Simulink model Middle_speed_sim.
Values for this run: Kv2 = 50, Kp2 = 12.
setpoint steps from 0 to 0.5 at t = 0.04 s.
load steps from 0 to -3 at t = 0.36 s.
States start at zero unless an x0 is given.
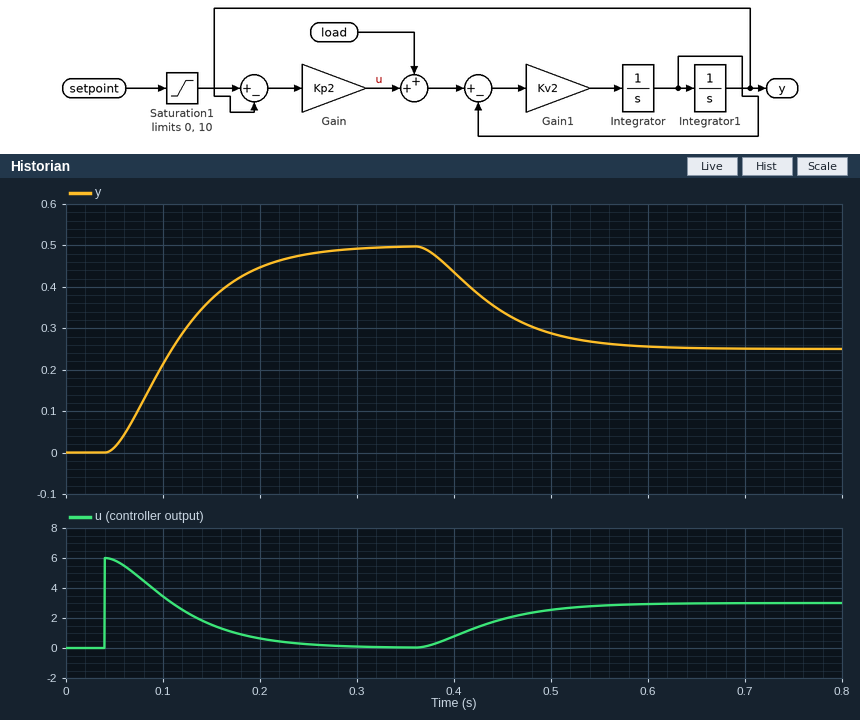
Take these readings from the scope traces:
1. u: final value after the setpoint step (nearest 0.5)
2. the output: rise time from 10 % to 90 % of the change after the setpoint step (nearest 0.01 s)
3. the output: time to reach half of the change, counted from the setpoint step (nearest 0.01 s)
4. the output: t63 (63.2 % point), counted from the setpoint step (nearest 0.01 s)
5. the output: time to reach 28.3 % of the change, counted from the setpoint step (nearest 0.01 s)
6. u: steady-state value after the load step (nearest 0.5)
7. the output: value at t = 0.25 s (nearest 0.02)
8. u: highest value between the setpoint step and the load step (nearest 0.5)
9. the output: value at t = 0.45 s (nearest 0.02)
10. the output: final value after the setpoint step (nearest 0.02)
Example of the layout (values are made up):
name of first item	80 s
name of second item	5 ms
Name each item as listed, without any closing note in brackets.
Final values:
u: final value after the setpoint step	0.0
the output: rise time from 10 % to 90 % of the change after the setpoint step	0.14 s
the output: time to reach half of the change, counted from the setpoint step	0.07 s
the output: t63 (63.2 % point), counted from the setpoint step	0.09 s
the output: time to reach 28.3 % of the change, counted from the setpoint step	0.04 s
u: steady-state value after the load step	3.0
the output: value at t = 0.25 s	0.48
u: highest value between the setpoint step and the load step	6.0
the output: value at t = 0.45 s	0.34
the output: final value after the setpoint step	0.50
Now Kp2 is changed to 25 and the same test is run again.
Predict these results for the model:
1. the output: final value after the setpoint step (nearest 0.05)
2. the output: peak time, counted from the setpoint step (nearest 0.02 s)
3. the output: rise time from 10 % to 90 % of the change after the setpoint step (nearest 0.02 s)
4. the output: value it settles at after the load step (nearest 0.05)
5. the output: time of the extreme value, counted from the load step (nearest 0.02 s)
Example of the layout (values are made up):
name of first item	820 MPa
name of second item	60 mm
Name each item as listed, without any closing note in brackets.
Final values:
the output: final value after the setpoint step	0.50
the output: peak time, counted from the setpoint step	0.12 s
the output: rise time from 10 % to 90 % of the change after the setpoint step	0.06 s
the output: value it settles at after the load step	0.40
the output: time of the extreme value, counted from the load step	0.12 s
